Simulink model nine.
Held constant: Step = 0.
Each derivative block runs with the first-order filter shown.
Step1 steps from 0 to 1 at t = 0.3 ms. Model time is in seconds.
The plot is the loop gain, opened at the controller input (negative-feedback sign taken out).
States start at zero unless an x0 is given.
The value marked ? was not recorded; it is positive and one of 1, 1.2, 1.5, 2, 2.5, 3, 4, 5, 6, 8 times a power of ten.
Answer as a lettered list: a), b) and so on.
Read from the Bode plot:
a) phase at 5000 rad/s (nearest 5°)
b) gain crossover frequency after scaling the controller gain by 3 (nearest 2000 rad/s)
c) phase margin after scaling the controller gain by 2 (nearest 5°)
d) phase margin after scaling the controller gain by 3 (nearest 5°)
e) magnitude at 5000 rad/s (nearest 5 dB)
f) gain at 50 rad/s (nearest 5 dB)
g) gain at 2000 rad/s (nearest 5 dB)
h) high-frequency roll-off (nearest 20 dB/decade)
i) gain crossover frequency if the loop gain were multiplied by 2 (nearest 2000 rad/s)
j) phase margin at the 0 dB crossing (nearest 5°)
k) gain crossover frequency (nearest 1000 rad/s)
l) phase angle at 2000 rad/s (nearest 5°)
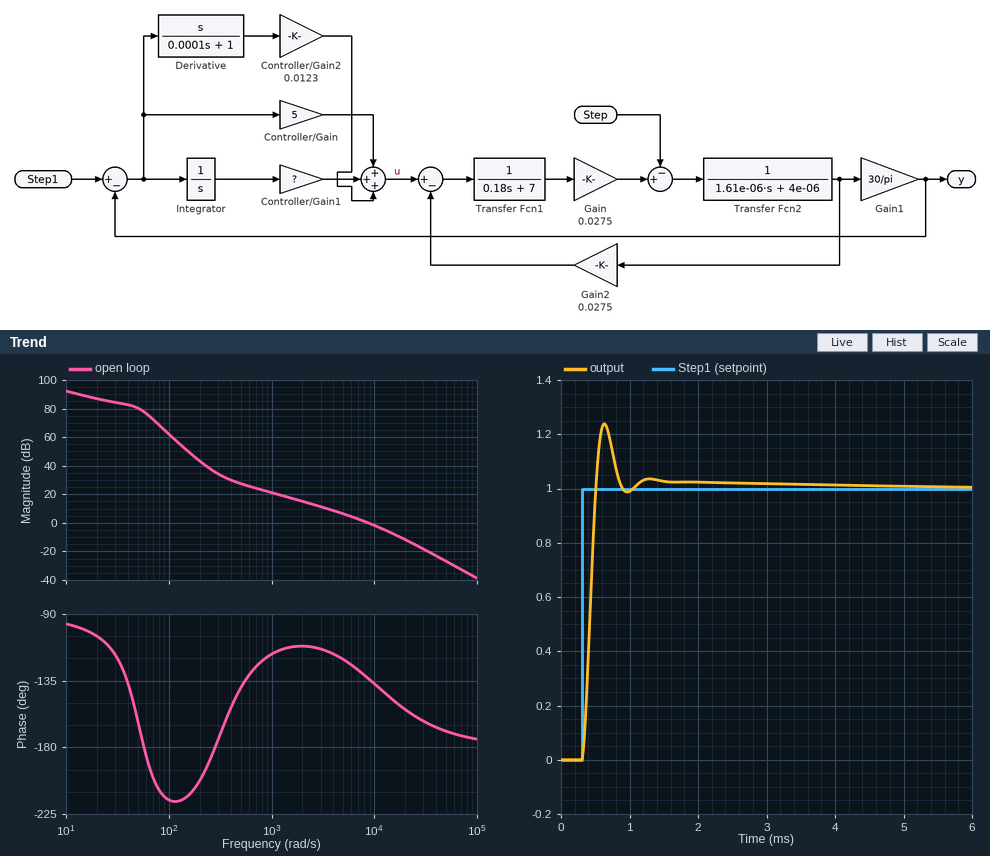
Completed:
a) -120°
b) 18000 rad/s
c) 35°
d) 30°
e) 5 dB
f) 80 dB
g) 15 dB
h) -40 dB/decade
i) 14000 rad/s
j) 45°
k) 9000 rad/s
l) -110°
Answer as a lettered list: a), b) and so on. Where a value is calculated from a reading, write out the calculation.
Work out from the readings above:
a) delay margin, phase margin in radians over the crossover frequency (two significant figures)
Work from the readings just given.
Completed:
a) 45 × π / 180 / 9000 = 0.000087 s
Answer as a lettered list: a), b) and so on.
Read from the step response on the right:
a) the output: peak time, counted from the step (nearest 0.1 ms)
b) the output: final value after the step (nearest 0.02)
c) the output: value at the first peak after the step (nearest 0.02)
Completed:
a) 0.3 ms
b) 1.00
c) 1.24
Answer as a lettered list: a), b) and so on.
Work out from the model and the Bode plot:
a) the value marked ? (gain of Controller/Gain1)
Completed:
a) 1200
